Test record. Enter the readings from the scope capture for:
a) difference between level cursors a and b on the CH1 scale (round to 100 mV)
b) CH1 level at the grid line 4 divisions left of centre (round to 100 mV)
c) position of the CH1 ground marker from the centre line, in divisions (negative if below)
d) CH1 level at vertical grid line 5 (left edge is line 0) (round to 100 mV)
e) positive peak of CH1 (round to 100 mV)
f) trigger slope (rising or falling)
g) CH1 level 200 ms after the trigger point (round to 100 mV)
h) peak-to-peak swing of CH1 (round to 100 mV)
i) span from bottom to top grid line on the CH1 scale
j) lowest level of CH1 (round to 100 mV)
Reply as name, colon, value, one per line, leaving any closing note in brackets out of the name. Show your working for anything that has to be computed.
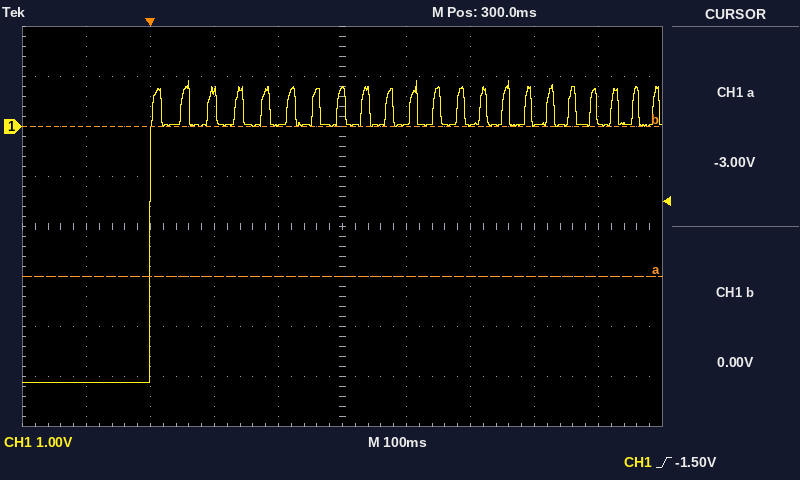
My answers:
difference between level cursors a and b on the CH1 scale: 3.0 V
CH1 level at the grid line 4 divisions left of centre: -5.1 V
position of the CH1 ground marker from the centre line, in divisions: +2.0 div
CH1 level at vertical grid line 5 (left edge is line 0): 700 mV
positive peak of CH1: 900 mV
trigger slope: rising
CH1 level 200 ms after the trigger point: 0.0 V
peak-to-peak swing of CH1: 900 mV − (-5.1 V) = 6.0 V
span from bottom to top grid line on the CH1 scale: 8 V
lowest level of CH1: -5.1 V
